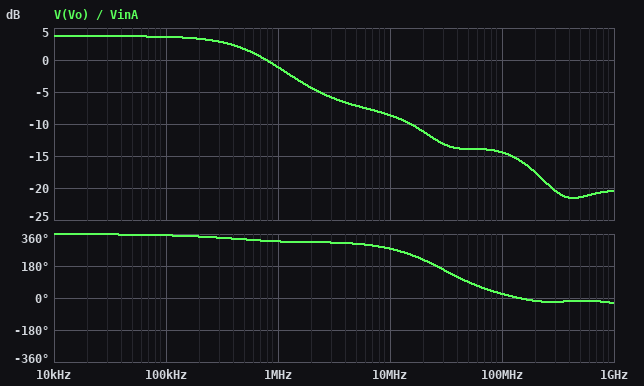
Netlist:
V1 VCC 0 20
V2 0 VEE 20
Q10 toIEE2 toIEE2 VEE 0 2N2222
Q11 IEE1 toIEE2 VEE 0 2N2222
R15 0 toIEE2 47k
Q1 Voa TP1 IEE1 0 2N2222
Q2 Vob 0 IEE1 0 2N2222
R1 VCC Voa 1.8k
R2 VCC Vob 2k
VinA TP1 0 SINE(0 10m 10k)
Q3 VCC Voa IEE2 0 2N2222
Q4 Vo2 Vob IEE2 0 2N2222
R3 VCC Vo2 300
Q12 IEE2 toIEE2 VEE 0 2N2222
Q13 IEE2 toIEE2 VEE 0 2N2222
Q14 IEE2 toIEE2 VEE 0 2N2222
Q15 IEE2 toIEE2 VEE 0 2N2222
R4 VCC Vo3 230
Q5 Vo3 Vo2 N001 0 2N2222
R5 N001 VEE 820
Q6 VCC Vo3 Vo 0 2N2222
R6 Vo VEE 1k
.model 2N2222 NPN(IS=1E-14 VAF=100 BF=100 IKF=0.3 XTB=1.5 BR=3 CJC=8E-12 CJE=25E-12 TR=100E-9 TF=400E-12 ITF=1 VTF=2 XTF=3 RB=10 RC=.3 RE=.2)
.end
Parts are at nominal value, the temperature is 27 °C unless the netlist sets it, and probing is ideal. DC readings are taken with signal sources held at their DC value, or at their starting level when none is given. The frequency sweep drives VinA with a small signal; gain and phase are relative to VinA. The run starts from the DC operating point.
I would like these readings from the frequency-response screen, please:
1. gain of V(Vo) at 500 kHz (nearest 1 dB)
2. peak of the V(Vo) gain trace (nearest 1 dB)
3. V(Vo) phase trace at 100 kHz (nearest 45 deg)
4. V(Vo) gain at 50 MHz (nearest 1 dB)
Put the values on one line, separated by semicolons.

2 dB; 4 dB; 360 deg; -14 dB
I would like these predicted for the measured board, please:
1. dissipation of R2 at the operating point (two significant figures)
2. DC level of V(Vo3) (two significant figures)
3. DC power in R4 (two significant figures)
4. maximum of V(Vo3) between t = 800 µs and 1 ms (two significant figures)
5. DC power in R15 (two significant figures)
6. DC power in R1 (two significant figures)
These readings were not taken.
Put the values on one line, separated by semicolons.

6.2 mW; 15 V; 120 mW; 15 V; 8.0 mW; 160 µW
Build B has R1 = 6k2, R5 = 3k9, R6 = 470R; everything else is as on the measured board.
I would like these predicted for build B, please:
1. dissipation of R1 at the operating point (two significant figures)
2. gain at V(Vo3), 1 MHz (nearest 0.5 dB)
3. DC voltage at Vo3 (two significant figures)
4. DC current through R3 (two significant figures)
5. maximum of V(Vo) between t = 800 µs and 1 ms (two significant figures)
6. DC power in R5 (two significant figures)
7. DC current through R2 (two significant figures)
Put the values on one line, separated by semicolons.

320 µW; -11.5 dB; 18 V; 4.2 mA; 17 V; 370 mW; 320 µA
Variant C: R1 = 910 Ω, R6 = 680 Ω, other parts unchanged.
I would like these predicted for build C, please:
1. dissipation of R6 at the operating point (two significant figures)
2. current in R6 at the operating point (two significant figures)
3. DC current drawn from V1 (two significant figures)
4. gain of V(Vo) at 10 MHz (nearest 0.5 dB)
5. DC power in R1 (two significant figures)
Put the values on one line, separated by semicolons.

1.7 W; 50 mA; 95 mA; -7.5 dB; 82 µW
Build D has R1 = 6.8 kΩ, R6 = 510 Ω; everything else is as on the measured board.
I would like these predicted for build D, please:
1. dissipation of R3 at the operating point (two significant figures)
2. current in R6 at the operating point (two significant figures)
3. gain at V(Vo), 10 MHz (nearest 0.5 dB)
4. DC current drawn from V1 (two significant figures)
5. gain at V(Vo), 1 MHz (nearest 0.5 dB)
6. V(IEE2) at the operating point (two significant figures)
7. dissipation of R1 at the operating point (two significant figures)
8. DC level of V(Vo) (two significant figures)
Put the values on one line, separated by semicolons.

61 mW; 67 mA; -8.0 dB; 110 mA; -2.0 dB; 17 V; 600 µW; 14 V
